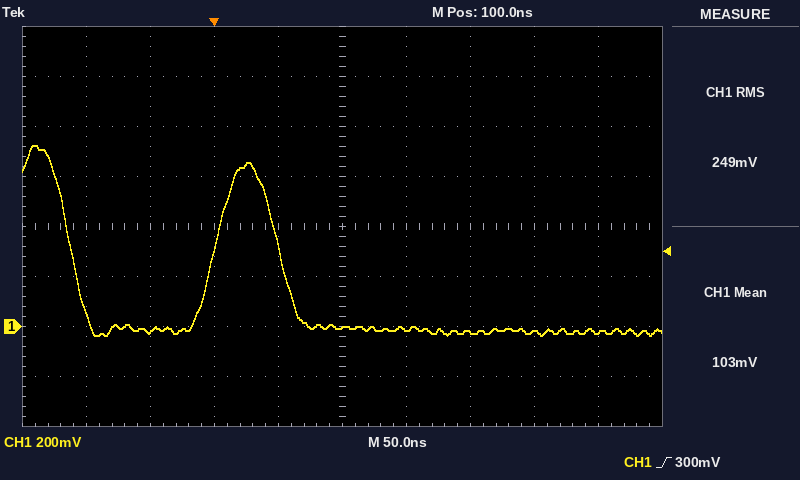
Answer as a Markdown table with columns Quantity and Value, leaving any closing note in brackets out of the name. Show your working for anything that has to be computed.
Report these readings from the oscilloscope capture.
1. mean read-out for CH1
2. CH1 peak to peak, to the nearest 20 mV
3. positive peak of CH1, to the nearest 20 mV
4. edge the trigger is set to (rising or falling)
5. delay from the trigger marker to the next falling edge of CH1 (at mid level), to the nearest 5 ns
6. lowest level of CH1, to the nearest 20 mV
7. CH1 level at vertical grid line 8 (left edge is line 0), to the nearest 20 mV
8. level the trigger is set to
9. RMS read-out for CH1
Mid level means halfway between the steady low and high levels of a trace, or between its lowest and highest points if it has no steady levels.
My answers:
| Quantity | Value |
|---|---|
| mean read-out for CH1 | 103 mV |
| CH1 peak to peak, to the nearest 20 mV | 720 mV − (-40 mV) = 760 mV |
| positive peak of CH1, to the nearest 20 mV | 720 mV |
| edge the trigger is set to | rising |
| delay from the trigger marker to the next falling edge of CH1 (at mid level), to the nearest 5 ns | 50 ns |
| lowest level of CH1, to the nearest 20 mV | -40 mV |
| CH1 level at vertical grid line 8 (left edge is line 0), to the nearest 20 mV | -20 mV |
| level the trigger is set to | 300 mV |
| RMS read-out for CH1 | 249 mV |
